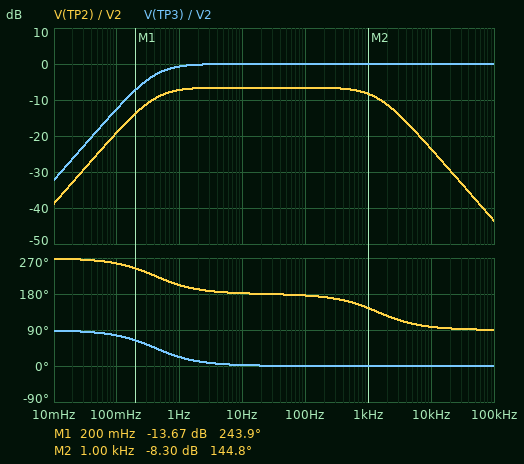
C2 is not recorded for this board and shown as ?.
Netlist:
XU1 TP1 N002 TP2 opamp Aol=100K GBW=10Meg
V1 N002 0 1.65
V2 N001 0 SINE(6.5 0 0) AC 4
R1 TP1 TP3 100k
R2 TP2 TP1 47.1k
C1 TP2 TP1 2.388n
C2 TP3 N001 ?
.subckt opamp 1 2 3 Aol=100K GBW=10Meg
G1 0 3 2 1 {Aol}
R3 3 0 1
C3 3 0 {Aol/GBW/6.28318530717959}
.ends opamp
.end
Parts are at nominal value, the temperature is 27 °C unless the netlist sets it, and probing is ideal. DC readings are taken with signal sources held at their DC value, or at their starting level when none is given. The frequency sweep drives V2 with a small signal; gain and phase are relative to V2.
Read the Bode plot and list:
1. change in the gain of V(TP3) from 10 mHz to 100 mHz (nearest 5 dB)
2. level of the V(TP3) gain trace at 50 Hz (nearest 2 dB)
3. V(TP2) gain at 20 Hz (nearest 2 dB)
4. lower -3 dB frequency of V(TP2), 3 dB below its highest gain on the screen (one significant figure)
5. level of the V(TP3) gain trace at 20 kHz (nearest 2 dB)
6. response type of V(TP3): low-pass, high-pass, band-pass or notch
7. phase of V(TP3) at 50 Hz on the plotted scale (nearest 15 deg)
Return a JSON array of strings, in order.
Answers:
["20 dB", "0 dB", "-6 dB", "400 mHz", "0 dB", "high-pass", "0 deg"]
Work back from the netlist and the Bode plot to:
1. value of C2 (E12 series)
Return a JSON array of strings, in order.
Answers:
["3.9 µF"]
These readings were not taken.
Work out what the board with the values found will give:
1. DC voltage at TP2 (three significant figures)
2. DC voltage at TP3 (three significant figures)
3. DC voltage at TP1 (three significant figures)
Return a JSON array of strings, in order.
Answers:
["1.65 V", "1.65 V", "1.65 V"]
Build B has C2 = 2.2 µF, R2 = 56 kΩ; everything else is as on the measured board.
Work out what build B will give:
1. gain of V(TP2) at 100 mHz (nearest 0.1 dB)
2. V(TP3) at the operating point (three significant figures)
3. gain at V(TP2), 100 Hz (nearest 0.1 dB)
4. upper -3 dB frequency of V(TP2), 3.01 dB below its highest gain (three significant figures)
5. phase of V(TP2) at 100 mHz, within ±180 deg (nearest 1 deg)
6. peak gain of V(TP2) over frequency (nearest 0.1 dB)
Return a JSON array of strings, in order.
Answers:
["-22.3 dB", "1.65 V", "-5.1 dB", "1.19 kHz", "-98 deg", "-5.0 dB"]
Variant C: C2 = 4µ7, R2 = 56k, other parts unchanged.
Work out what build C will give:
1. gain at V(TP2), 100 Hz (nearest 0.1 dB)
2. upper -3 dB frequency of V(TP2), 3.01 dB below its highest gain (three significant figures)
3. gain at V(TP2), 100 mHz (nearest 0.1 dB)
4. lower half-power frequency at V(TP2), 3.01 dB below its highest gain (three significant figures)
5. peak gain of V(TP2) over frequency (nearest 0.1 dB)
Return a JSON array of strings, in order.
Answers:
["-5.1 dB", "1.19 kHz", "-16.0 dB", "338 mHz", "-5.0 dB"]
